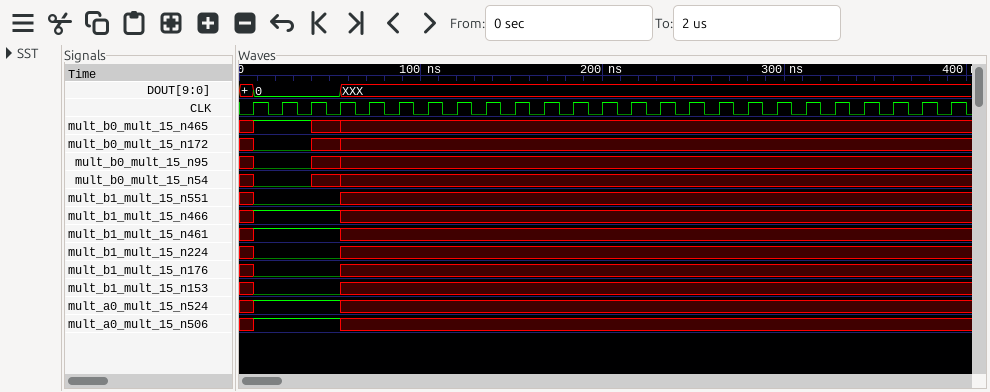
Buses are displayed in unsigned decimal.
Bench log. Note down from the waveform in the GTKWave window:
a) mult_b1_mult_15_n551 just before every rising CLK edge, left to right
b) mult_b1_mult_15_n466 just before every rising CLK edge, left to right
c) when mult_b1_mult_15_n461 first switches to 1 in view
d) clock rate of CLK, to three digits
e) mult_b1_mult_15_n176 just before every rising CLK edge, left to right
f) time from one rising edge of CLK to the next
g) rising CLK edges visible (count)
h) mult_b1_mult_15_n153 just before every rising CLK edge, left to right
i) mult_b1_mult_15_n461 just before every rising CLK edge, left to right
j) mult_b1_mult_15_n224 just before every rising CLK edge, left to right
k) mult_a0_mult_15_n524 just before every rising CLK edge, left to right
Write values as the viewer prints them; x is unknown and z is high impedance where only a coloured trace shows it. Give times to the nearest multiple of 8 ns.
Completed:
x 0 0 0 x x x x x x x x x x x x x x x x x x x x x
x 1 1 1 x x x x x x x x x x x x x x x x x x x x x
8 ns
62.5 MHz
x 0 0 0 x x x x x x x x x x x x x x x x x x x x x
16 ns
25
x 0 0 0 x x x x x x x x x x x x x x x x x x x x x
x 1 1 1 x x x x x x x x x x x x x x x x x x x x x
x 0 0 0 x x x x x x x x x x x x x x x x x x x x x
x 1 1 1 x x x x x x x x x x x x x x x x x x x x x
